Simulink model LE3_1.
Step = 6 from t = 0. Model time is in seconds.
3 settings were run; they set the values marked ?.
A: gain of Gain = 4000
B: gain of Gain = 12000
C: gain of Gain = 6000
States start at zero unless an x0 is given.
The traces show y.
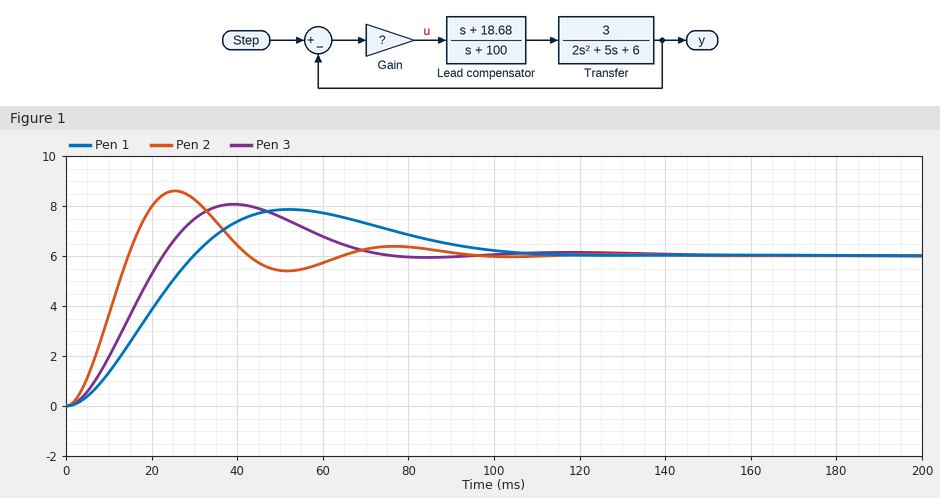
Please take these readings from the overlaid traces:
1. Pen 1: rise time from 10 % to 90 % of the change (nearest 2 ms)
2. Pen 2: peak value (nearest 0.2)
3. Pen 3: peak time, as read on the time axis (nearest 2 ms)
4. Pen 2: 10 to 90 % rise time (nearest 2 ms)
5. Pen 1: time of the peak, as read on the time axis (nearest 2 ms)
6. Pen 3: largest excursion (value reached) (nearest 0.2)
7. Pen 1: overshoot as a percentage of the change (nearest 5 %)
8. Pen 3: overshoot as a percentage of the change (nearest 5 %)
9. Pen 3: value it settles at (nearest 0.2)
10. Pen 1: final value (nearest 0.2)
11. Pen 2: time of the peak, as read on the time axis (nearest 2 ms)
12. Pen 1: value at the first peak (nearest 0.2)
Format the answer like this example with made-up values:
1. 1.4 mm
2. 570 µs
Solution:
1. 20 ms
2. 8.6
3. 40 ms
4. 10 ms
5. 52 ms
6. 8.0
7. 30 %
8. 35 %
9. 6.0
10. 6.0
11. 26 ms
12. 7.8
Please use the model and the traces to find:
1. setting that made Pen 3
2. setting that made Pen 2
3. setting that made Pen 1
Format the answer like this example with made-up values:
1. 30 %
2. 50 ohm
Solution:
1. C
2. B
3. A
